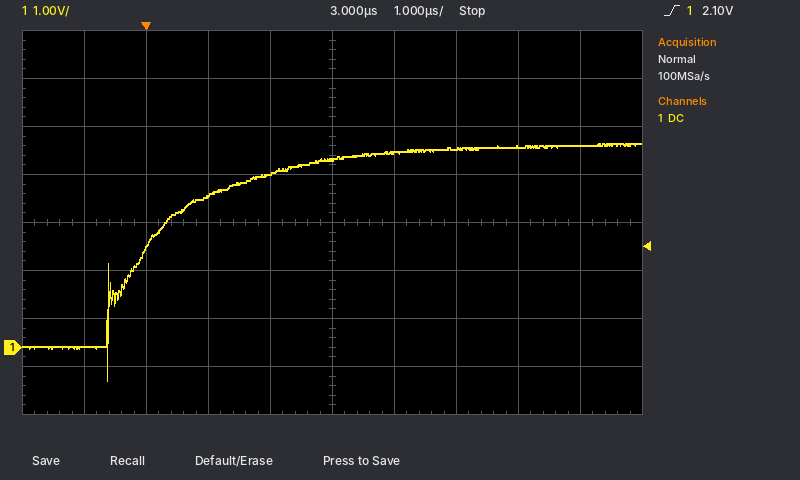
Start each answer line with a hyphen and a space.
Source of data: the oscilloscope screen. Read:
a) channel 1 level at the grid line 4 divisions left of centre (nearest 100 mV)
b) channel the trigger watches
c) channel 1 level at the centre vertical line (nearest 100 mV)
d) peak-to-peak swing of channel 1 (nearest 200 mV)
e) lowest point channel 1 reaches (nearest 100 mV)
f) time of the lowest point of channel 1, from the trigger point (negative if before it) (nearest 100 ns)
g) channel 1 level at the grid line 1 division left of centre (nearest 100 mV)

- 0.0 V
- channel 1
- 3.9 V
- 5.0 V
- -700 mV
- -600 ns
- 3.6 V
